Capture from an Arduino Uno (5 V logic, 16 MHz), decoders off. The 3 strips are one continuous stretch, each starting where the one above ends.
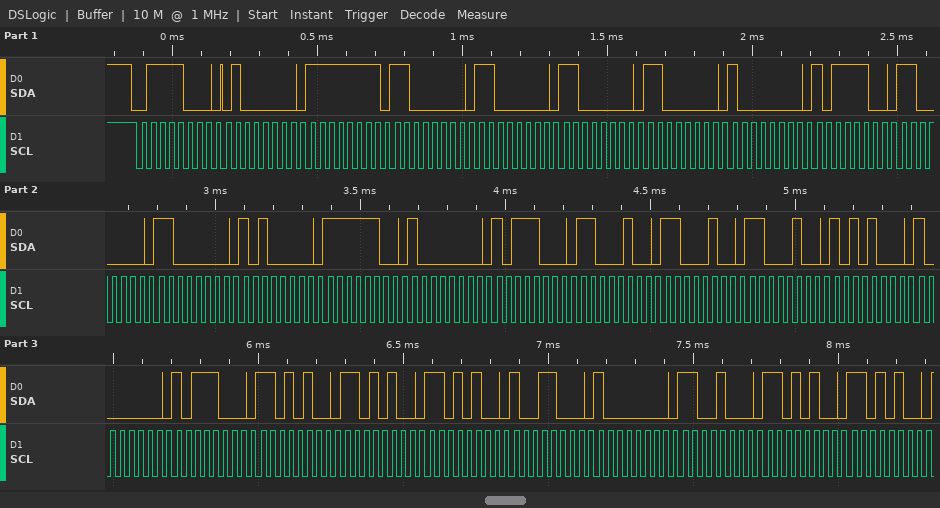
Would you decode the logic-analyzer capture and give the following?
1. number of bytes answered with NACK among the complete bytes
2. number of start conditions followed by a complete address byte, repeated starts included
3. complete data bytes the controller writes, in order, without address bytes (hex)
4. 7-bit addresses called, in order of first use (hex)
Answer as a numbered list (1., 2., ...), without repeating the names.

1. 0
2. 1
3. 40 FF C0 C0 C0 C0 80 BC C0 C0 A0 FC 80 B8 C4 C4 C4 A8 80 B8 D4 D4 D4 98 80 C8 D4 D4
4. 0x3C
